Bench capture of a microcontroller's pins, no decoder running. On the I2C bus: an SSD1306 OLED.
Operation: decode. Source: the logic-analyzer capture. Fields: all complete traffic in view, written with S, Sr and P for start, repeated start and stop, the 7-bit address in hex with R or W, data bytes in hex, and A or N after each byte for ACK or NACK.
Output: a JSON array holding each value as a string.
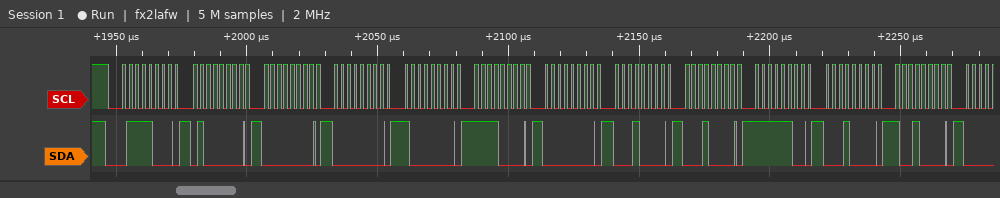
["S 3CW A 40 A 00 A 00 A 80 A F0 A 00 A 10 A 10 A FC A 10 A 90 A"]
